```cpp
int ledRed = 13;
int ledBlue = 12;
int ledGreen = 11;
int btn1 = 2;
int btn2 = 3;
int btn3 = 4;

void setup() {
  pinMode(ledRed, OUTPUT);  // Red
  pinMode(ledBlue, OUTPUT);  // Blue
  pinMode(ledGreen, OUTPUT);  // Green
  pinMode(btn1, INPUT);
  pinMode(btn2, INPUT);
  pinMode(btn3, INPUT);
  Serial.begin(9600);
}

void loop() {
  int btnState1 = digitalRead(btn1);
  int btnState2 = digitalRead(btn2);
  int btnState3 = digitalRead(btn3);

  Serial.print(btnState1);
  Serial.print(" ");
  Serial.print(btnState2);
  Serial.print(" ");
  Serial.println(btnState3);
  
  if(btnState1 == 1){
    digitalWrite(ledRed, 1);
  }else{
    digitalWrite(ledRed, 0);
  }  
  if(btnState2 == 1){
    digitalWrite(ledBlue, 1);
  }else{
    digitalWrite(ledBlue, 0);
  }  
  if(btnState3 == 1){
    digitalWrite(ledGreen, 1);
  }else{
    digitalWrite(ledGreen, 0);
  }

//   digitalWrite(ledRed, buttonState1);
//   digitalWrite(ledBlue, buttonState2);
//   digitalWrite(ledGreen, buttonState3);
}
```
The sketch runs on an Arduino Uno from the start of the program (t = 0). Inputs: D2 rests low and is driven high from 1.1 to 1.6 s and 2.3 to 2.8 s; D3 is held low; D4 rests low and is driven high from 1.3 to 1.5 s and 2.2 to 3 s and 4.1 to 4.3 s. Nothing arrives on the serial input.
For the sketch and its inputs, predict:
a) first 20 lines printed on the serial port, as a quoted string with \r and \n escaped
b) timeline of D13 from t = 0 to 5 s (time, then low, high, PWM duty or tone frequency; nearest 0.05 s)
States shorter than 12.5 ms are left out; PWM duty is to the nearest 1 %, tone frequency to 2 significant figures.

"0 0 0\r\n0 0 0\r\n0 0 0\r\n0 0 0\r\n0 0 0\r\n0 0 0\r\n0 0 0\r\n0 0 0\r\n0 0 0\r\n0 0 0\r\n0 0 0\r\n0 0 0\r\n0 0 0\r\n0 0 0\r\n0 0 0\r\n0 0 0\r\n0 0 0\r\n0 0 0\r\n0 0 0\r\n0 0 0\r\n"
0 s low; 1.1 s high; 1.6 s low; 2.3 s high; 2.8 s low
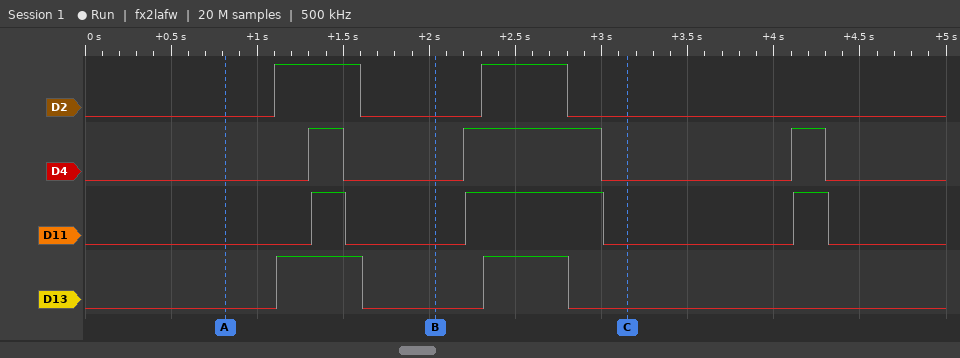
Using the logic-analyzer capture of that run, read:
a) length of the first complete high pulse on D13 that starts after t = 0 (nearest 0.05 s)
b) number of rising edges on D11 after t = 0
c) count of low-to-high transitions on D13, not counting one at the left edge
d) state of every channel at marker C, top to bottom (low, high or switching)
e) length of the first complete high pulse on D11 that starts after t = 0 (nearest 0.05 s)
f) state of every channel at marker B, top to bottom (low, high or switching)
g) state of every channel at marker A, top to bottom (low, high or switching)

0.50 s
3
2
D2 low, D4 low, D11 low, D13 low
0.20 s
D2 low, D4 low, D11 low, D13 low
D2 low, D4 low, D11 low, D13 low
